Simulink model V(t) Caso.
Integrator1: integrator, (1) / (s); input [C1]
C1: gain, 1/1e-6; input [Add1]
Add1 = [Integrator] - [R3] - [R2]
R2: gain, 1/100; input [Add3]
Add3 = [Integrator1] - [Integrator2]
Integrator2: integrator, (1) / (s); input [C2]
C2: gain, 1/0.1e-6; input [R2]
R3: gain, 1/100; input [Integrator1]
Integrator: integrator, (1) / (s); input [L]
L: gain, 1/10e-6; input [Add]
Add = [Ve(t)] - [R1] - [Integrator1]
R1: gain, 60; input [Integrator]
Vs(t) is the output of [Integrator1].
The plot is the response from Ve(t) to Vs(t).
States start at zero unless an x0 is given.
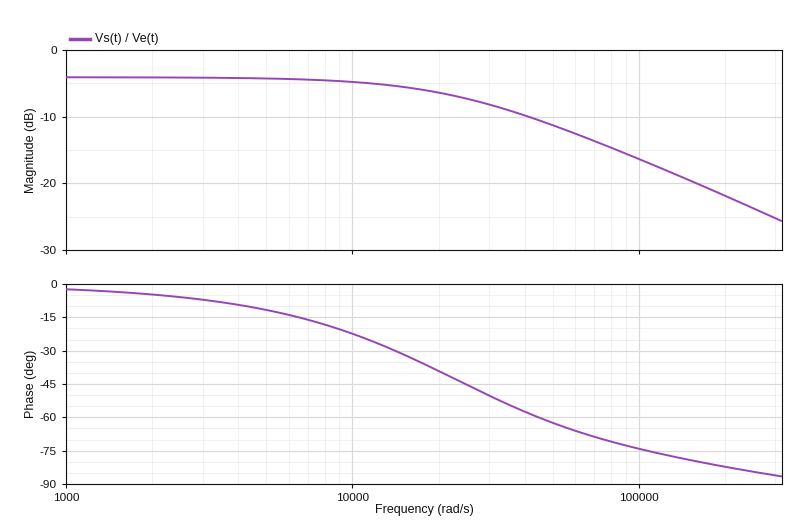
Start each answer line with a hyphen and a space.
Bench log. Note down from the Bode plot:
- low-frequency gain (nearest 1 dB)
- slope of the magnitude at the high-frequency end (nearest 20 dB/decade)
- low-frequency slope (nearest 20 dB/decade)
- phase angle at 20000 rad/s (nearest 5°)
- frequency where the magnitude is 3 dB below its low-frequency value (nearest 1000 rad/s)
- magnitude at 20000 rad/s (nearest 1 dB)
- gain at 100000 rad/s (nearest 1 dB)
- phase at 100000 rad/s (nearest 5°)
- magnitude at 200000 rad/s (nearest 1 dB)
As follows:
- -4 dB
- -20 dB/decade
- 0 dB/decade
- -40°
- 24000 rad/s
- -6 dB
- -16 dB
- -75°
- -22 dB
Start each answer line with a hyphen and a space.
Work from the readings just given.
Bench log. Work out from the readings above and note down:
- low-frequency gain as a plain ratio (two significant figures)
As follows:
- 0.63
